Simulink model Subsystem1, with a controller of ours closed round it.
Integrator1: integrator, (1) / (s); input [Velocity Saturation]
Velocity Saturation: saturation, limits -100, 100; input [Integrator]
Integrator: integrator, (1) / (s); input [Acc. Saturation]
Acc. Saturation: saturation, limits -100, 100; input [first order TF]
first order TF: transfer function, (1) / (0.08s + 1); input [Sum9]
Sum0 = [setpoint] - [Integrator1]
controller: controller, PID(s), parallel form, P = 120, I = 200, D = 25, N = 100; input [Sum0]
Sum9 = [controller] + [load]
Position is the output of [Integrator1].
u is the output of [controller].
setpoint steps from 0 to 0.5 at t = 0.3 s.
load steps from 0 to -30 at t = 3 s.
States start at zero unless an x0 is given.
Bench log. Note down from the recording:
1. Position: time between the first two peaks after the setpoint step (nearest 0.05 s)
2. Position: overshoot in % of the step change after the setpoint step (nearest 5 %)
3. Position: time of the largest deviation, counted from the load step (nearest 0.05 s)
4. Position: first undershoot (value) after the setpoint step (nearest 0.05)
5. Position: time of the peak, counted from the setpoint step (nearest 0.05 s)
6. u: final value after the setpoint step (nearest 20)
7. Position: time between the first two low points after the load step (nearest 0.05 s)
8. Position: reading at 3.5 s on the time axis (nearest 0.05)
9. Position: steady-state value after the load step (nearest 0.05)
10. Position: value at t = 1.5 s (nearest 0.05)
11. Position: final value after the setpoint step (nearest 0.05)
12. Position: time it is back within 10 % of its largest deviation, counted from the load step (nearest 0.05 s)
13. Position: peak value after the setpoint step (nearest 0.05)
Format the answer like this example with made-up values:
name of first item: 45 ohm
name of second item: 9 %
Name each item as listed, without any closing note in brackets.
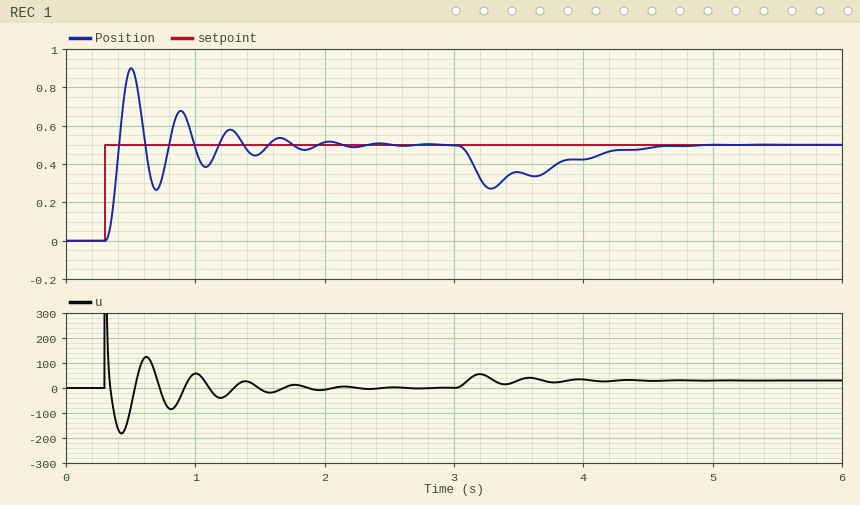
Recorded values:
Position: time between the first two peaks after the setpoint step: 0.40 s
Position: overshoot in % of the step change after the setpoint step: 80 %
Position: time of the largest deviation, counted from the load step: 0.30 s
Position: first undershoot (value) after the setpoint step: 0.25
Position: time of the peak, counted from the setpoint step: 0.20 s
u: final value after the setpoint step: 0
Position: time between the first two low points after the load step: 0.35 s
Position: reading at 3.5 s on the time axis: 0.35
Position: steady-state value after the load step: 0.50
Position: value at t = 1.5 s: 0.45
Position: final value after the setpoint step: 0.50
Position: time it is back within 10 % of its largest deviation, counted from the load step: 1.45 s
Position: peak value after the setpoint step: 0.90
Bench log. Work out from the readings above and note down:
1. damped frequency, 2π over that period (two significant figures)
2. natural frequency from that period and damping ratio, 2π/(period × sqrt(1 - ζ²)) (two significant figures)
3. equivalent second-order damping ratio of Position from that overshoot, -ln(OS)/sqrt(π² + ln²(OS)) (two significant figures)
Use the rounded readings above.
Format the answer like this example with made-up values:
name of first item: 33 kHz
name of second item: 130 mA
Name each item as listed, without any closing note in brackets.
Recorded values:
damped frequency, 2π over that period: 16 rad/s
natural frequency from that period and damping ratio, 2π/(period × sqrt(1 - ζ²)): 16 rad/s
equivalent second-order damping ratio of Position from that overshoot, -ln(OS)/sqrt(π² + ln²(OS)): 0.071
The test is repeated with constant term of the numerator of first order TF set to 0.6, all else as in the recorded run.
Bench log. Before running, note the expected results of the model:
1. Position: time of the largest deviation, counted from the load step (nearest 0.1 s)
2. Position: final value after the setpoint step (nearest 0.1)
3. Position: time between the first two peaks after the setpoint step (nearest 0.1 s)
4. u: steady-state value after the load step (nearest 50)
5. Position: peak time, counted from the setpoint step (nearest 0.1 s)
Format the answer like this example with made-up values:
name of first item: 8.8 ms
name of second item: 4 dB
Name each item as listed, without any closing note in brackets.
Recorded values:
Position: time of the largest deviation, counted from the load step: 0.4 s
Position: final value after the setpoint step: 0.5
Position: time between the first two peaks after the setpoint step: 0.5 s
u: steady-state value after the load step: 50
Position: peak time, counted from the setpoint step: 0.3 s
